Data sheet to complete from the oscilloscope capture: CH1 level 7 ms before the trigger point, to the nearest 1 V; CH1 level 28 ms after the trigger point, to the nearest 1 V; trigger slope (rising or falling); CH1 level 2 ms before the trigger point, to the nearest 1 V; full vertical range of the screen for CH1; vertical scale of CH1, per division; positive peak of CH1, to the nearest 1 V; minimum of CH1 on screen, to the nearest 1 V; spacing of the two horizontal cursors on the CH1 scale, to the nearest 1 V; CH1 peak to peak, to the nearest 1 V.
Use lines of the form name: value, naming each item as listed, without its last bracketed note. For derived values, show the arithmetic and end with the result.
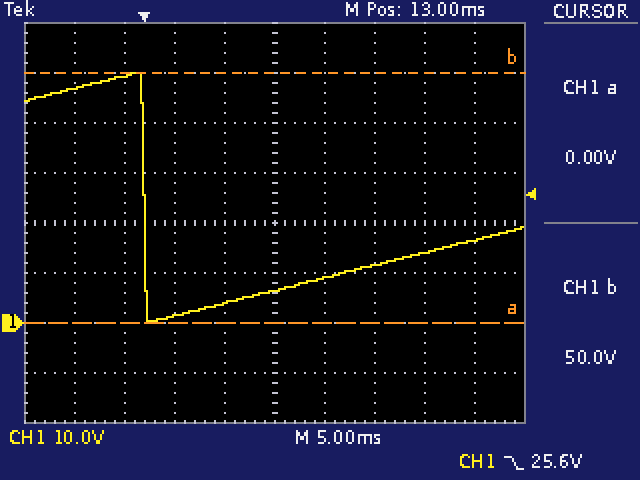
CH1 level 7 ms before the trigger point, to the nearest 1 V: 47 V
CH1 level 28 ms after the trigger point, to the nearest 1 V: 14 V
trigger slope: falling
CH1 level 2 ms before the trigger point, to the nearest 1 V: 49 V
full vertical range of the screen for CH1: 80 V
vertical scale of CH1, per division: 10 V
positive peak of CH1, to the nearest 1 V: 50 V
minimum of CH1 on screen, to the nearest 1 V: 0 V
spacing of the two horizontal cursors on the CH1 scale, to the nearest 1 V: 50 V
CH1 peak to peak, to the nearest 1 V: 50 V − (0 V) = 50 V
